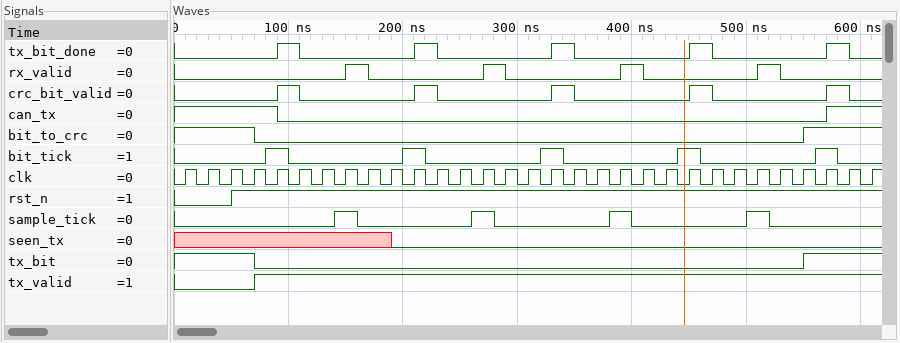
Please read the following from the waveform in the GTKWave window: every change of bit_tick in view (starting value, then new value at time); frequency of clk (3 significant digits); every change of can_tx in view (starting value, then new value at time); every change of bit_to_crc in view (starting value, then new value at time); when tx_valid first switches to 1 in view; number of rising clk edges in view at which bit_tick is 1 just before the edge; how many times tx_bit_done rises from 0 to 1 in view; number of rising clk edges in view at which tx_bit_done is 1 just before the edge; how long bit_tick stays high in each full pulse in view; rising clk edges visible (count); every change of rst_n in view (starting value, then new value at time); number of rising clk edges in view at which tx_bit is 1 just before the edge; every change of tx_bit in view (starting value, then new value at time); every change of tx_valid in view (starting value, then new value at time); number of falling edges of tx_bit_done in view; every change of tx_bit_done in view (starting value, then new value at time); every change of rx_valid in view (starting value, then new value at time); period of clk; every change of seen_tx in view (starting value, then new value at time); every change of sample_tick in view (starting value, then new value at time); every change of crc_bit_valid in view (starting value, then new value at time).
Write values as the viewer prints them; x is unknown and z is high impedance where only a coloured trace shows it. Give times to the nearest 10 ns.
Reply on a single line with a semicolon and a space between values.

0, 1 at 80 ns, 0 at 100 ns, 1 at 200 ns, 0 at 220 ns, 1 at 320 ns, 0 at 340 ns, 1 at 440 ns, 0 at 460 ns, 1 at 560 ns, 0 at 580 ns; 50.0 MHz; 1, 0 at 90 ns, 1 at 570 ns; 1, 0 at 70 ns, 1 at 550 ns; 70 ns; 5; 5; 5; 20 ns, 20 ns, 20 ns, 20 ns, 20 ns; 31; 0, 1 at 50 ns; 7; 1, 0 at 70 ns, 1 at 550 ns; 0, 1 at 70 ns; 5; 0, 1 at 90 ns, 0 at 110 ns, 1 at 210 ns, 0 at 230 ns, 1 at 330 ns, 0 at 350 ns, 1 at 450 ns, 0 at 470 ns, 1 at 570 ns, 0 at 590 ns; 0, 1 at 150 ns, 0 at 170 ns, 1 at 270 ns, 0 at 290 ns, 1 at 390 ns, 0 at 410 ns, 1 at 510 ns, 0 at 530 ns; 20 ns; x, 0 at 190 ns; 0, 1 at 140 ns, 0 at 160 ns, 1 at 260 ns, 0 at 280 ns, 1 at 380 ns, 0 at 400 ns, 1 at 500 ns, 0 at 520 ns; 0, 1 at 90 ns, 0 at 110 ns, 1 at 210 ns, 0 at 230 ns, 1 at 330 ns, 0 at 350 ns, 1 at 450 ns, 0 at 470 ns, 1 at 570 ns, 0 at 590 ns
